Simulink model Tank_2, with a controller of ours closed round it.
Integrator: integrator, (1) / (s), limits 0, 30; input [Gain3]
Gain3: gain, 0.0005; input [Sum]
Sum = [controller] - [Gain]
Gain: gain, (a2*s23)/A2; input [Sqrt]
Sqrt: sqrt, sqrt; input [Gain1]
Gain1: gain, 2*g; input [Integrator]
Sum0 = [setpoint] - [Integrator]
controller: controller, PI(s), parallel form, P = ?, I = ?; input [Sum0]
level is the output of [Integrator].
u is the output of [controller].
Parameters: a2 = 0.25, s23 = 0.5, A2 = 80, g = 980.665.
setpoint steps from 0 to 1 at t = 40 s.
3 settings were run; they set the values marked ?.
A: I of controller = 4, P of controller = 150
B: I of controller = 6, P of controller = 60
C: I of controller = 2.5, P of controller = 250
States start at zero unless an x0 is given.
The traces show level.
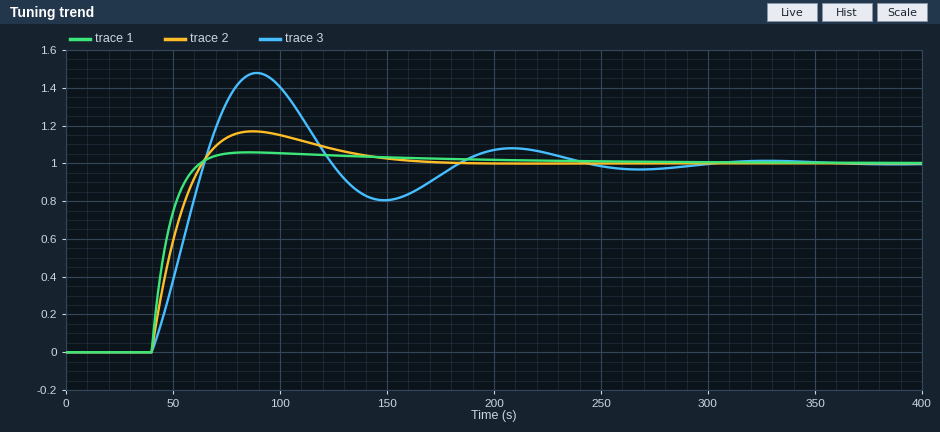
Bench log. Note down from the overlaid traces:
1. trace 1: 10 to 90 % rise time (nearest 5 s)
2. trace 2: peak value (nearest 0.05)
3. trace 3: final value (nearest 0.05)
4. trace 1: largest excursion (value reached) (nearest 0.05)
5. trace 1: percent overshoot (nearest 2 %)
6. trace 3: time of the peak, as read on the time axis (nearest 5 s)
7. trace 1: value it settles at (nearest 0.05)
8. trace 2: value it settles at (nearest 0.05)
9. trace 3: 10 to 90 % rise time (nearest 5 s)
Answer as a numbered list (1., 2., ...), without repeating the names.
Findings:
1. 15 s
2. 1.15
3. 1.00
4. 1.05
5. 6 %
6. 90 s
7. 1.00
8. 1.00
9. 20 s
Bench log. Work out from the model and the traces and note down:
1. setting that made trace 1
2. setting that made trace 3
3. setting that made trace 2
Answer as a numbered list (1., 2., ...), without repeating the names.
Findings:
1. C
2. B
3. A
